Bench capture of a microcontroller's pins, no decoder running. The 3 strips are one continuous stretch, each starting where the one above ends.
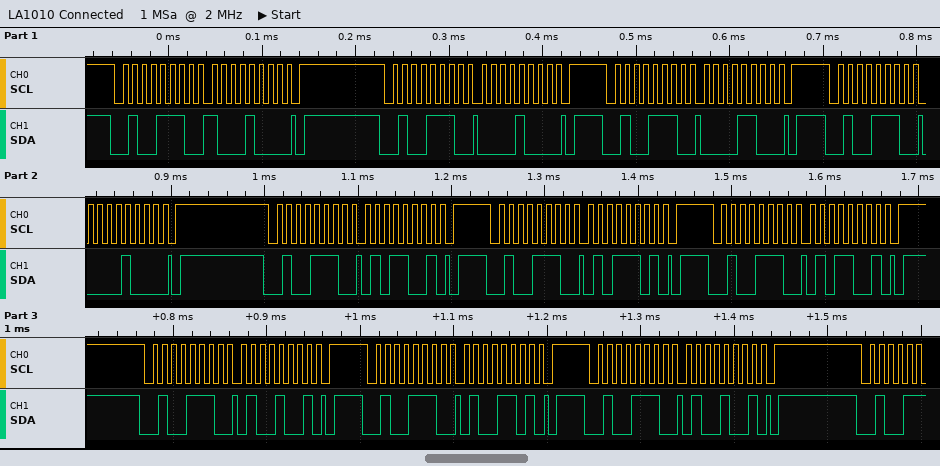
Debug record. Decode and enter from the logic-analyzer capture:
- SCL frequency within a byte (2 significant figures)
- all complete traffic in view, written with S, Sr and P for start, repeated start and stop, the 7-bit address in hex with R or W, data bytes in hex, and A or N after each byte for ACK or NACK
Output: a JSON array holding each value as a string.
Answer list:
["100 kHz", "S 27W A 88 A P S 27W A 08 A P S 27W A 0C A P S 27W A 08 A P S 27W A 59 A P S 27W A 5D A P S 27W A 59 A P S 27W A 49 A P S 27W A 4D A P S 27W A 49 A P"]
